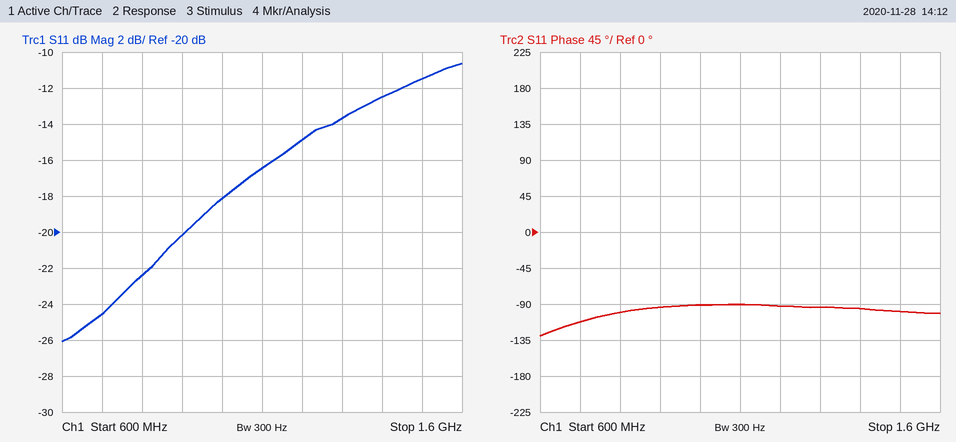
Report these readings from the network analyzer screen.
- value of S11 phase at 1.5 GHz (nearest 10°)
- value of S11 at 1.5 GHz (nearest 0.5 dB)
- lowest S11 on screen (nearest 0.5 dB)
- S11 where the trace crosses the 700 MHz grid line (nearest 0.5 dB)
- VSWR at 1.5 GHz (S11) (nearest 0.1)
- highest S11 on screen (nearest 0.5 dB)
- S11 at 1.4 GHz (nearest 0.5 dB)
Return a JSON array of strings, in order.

["-100°", "-11.5 dB", "-26.0 dB", "-24.5 dB", "1.7", "-10.5 dB", "-12.5 dB"]
